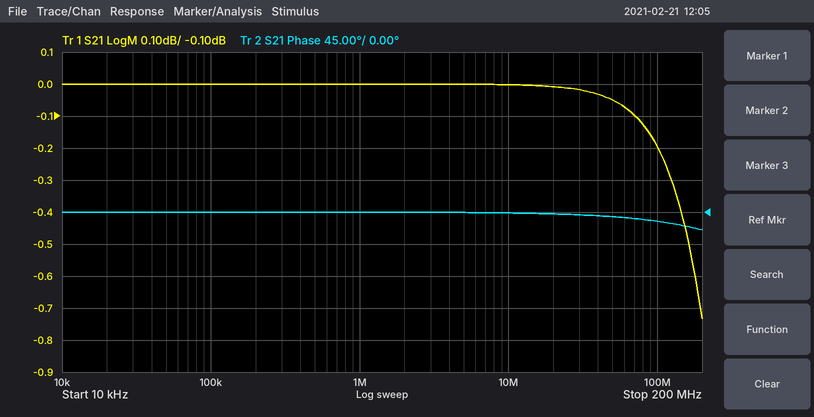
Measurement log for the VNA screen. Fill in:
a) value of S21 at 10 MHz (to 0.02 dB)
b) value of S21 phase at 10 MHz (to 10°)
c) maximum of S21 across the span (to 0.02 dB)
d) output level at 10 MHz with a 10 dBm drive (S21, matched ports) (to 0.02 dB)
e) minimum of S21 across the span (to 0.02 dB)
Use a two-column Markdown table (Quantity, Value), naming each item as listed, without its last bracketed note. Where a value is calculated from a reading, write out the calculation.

| Quantity | Value |
|---|---|
| value of S21 at 10 MHz | 0.00 dB |
| value of S21 phase at 10 MHz | 0° |
| maximum of S21 across the span | 0.00 dB |
| output level at 10 MHz with a 10 dBm drive (S21, matched ports) | 10 dBm + (0.00 dB) = 10.00 dBm |
| minimum of S21 across the span | -0.74 dB |
